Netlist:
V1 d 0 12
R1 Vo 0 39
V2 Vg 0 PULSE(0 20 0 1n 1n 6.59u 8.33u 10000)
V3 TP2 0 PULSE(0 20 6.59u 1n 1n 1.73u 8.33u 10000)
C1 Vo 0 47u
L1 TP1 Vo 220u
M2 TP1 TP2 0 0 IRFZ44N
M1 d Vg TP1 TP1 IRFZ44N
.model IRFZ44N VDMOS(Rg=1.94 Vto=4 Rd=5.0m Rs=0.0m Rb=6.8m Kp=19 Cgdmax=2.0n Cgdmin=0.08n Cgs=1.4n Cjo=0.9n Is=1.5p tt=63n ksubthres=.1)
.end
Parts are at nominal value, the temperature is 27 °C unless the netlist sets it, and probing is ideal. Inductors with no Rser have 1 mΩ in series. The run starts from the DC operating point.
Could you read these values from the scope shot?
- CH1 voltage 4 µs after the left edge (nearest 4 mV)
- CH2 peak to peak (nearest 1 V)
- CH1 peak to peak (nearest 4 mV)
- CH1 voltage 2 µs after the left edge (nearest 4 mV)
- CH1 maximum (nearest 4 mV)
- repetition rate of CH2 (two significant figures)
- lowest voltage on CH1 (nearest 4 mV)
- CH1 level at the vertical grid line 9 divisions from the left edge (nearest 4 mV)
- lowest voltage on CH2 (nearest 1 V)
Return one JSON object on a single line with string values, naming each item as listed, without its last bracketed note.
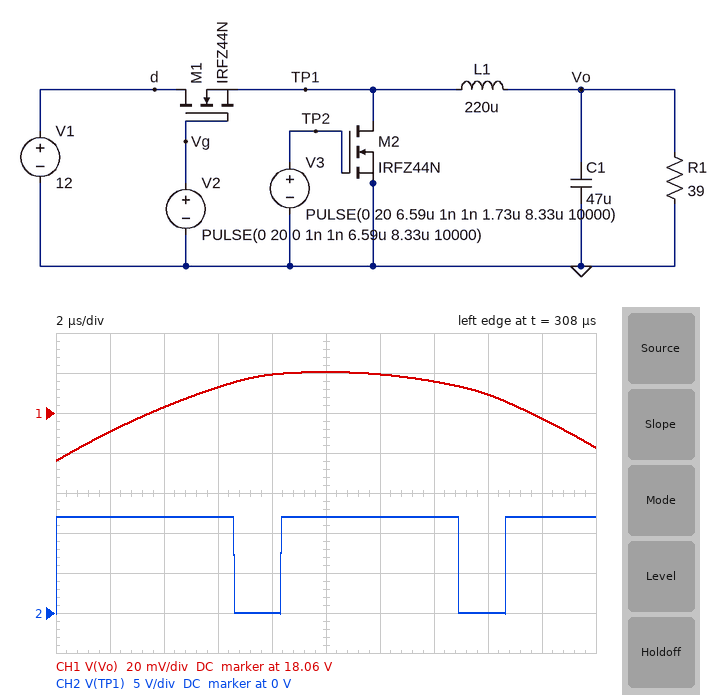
{"CH1 voltage 4 µs after the left edge": "18.064 V", "CH2 peak to peak": "12 V", "CH1 peak to peak": "44 mV", "CH1 voltage 2 µs after the left edge": "18.052 V", "CH1 maximum": "18.080 V", "repetition rate of CH2": "120 kHz", "lowest voltage on CH1": "18.036 V", "CH1 level at the vertical grid line 9 divisions from the left edge": "18.056 V", "lowest voltage on CH2": "0 V"}
